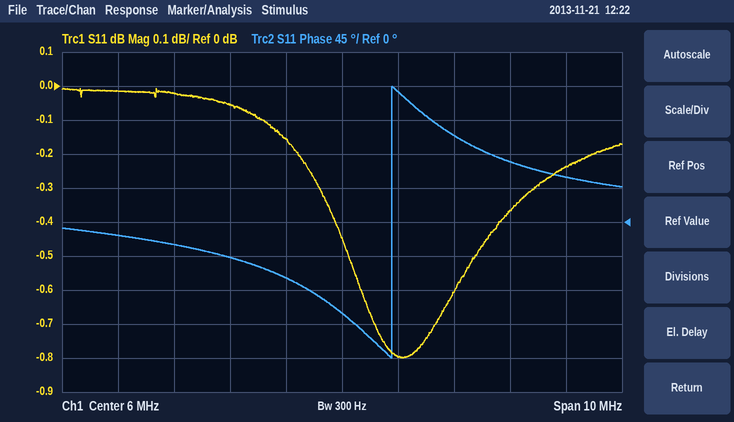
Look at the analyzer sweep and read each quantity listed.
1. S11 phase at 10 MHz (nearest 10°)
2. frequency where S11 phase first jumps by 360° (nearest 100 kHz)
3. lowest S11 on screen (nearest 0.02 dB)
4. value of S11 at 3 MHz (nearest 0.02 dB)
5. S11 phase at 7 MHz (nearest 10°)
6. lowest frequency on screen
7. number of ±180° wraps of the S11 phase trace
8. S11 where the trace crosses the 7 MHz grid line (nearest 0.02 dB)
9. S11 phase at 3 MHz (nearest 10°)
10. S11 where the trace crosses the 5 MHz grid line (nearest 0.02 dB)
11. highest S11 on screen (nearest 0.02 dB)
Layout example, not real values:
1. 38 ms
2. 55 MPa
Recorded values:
1. 60°
2. 6.9 MHz
3. -0.80 dB
4. -0.02 dB
5. 170°
6. 1 MHz
7. 1
8. -0.80 dB
9. -30°
10. -0.16 dB
11. 0.00 dB
